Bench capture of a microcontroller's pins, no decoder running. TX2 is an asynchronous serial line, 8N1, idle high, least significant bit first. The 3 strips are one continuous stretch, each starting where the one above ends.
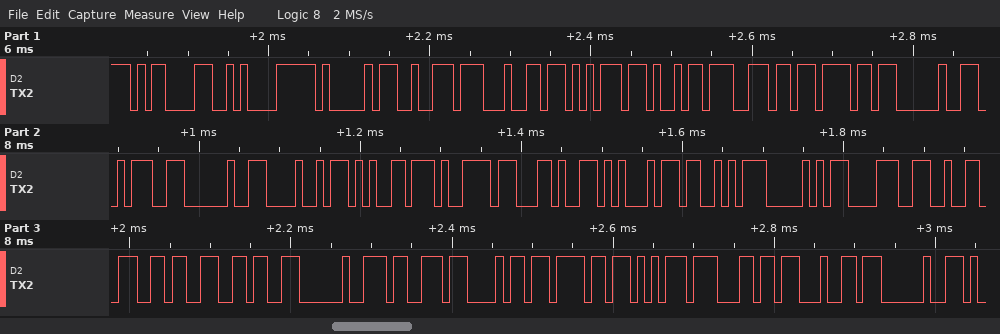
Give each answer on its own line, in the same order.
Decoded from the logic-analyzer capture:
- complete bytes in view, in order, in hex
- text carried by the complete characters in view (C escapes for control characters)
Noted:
0x0D 0x0A 0x41 0x72 0x64 0x75 0x69 0x6E 0x6F 0x20 0x3A 0x20 0x48 0x65 0x79 0x2C 0x45 0x53 0x50 0x38 0x32 0x36 0x36 0x20 0x73 0x68 0x6F 0x75 0x6C 0x64 0x20
"\r\nArduino : Hey,ESP8266 should "
